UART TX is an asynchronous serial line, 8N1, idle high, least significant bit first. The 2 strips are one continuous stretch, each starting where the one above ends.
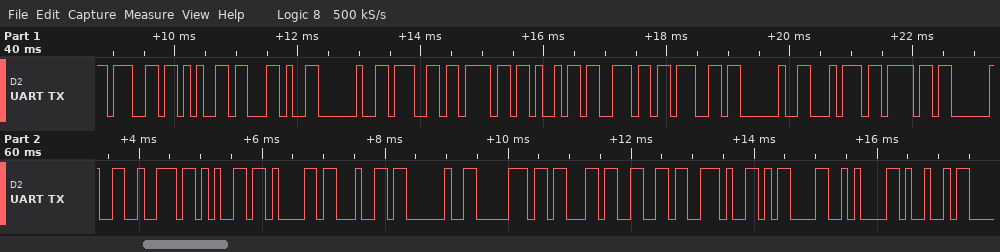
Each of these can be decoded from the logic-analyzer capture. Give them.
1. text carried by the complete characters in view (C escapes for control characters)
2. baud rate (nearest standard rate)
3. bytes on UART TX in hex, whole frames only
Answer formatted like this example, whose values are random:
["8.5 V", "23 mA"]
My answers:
["\"ge, going to read pcf.\\r\\nI\"", "9600 baud", "67 65 2C 20 67 6F 69 6E 67 20 74 6F 20 72 65 61 64 20 70 63 66 2E 0D 0A 49"]
